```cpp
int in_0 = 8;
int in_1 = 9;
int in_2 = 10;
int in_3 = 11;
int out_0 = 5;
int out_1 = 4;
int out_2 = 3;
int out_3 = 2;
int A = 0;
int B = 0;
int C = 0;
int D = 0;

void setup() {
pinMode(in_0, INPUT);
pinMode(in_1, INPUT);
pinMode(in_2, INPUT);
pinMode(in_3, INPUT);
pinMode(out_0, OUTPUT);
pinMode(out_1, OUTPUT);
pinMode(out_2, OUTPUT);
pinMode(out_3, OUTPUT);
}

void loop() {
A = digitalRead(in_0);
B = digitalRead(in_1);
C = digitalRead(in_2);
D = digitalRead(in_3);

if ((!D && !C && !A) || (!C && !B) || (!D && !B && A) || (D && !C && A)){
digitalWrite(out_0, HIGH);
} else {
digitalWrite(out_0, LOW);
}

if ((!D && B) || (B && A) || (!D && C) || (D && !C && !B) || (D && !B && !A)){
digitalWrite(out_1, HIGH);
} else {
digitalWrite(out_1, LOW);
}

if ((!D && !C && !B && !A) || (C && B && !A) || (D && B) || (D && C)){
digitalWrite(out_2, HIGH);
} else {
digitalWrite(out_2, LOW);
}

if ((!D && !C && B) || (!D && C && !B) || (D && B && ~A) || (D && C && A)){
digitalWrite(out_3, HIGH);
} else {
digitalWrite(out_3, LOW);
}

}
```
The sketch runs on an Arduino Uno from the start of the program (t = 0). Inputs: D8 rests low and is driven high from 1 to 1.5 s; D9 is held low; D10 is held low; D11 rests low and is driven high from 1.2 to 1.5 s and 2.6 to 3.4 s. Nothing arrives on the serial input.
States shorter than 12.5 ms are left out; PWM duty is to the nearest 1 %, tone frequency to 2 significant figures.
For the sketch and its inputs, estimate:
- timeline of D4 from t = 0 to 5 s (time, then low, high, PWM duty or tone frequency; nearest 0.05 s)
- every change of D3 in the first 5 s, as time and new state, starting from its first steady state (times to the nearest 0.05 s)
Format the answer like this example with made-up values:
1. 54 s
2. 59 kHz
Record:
1. 0 s low; 1.2 s high; 1.5 s low; 2.6 s high; 3.4 s low
2. 0 s high; 1 s low; 1.5 s high; 2.6 s low; 3.4 s high
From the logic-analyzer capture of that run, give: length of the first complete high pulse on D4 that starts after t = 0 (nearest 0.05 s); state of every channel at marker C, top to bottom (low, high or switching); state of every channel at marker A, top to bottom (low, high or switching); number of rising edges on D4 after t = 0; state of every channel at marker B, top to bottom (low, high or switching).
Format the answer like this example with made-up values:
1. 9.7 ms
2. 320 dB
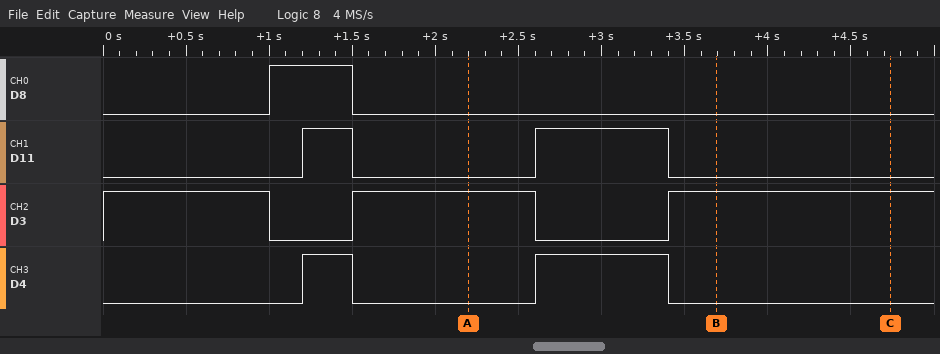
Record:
1. 0.30 s
2. D8 low, D11 low, D3 high, D4 low
3. D8 low, D11 low, D3 high, D4 low
4. 2
5. D8 low, D11 low, D3 high, D4 low
